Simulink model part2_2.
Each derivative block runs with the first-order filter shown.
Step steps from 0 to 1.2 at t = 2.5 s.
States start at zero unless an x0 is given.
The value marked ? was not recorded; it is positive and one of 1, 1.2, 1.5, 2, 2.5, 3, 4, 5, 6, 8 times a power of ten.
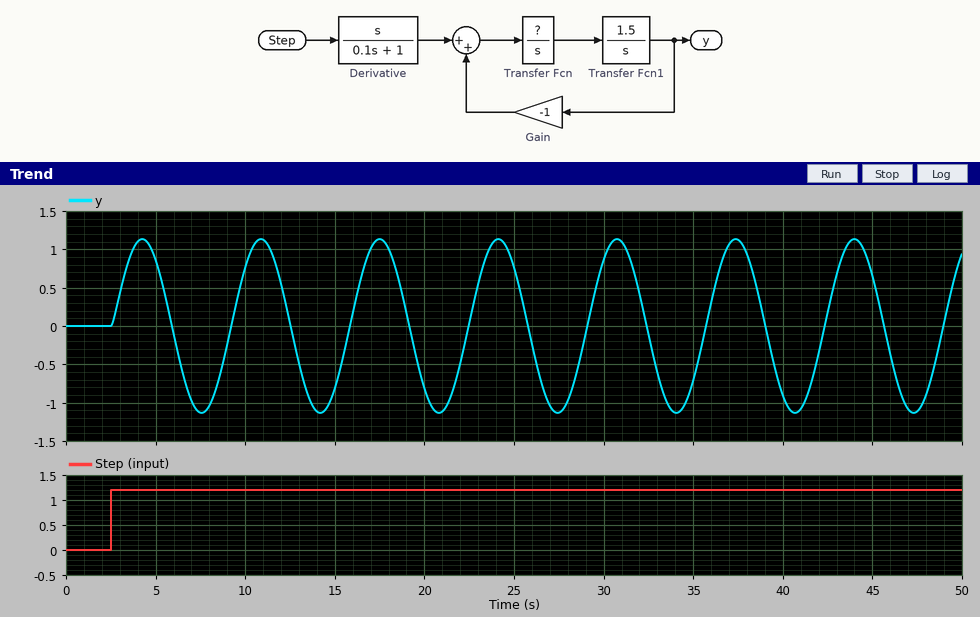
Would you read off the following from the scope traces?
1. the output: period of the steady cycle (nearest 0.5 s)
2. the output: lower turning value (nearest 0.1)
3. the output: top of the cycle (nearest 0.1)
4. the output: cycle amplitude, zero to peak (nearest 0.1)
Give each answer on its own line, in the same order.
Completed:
6.5 s
-1.1
1.1
1.1
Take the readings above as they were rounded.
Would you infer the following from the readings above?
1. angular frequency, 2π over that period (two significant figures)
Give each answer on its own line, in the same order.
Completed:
0.97 rad/s
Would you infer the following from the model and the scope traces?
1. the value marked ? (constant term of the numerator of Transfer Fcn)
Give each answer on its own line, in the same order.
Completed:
0.6
